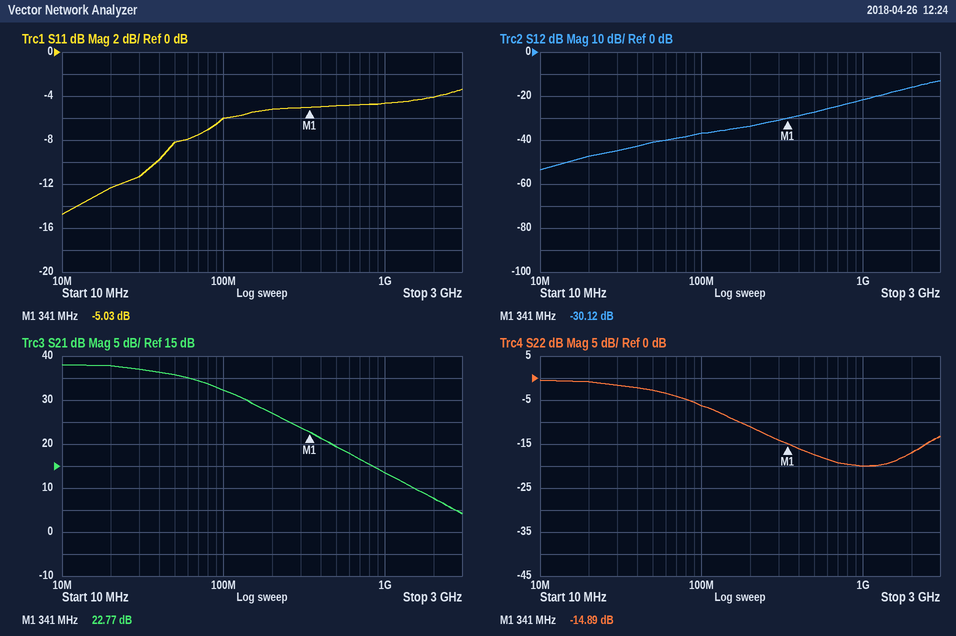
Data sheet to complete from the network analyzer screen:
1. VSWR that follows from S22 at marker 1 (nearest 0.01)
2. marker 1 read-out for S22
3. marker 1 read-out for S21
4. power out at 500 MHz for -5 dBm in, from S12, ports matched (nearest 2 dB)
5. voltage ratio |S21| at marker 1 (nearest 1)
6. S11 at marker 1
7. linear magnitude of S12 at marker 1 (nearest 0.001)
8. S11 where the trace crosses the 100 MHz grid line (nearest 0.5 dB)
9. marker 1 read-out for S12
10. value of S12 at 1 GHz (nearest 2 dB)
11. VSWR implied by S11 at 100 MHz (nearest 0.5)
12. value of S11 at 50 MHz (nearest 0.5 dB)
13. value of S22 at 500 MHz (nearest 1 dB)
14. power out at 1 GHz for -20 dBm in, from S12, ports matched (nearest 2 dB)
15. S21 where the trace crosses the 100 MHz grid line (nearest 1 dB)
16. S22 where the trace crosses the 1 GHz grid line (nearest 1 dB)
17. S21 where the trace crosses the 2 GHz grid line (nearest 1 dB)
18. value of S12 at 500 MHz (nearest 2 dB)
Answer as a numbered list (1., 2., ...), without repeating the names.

1. 1.44
2. -14.89 dB
3. 22.77 dB
4. -32 dBm
5. 14
6. -5.03 dB
7. 0.031
8. -6.0 dB
9. -30.12 dB
10. -22 dB
11. 3.0
12. -8.0 dB
13. -17 dB
14. -42 dBm
15. 32 dB
16. -20 dB
17. 8 dB
18. -28 dB
